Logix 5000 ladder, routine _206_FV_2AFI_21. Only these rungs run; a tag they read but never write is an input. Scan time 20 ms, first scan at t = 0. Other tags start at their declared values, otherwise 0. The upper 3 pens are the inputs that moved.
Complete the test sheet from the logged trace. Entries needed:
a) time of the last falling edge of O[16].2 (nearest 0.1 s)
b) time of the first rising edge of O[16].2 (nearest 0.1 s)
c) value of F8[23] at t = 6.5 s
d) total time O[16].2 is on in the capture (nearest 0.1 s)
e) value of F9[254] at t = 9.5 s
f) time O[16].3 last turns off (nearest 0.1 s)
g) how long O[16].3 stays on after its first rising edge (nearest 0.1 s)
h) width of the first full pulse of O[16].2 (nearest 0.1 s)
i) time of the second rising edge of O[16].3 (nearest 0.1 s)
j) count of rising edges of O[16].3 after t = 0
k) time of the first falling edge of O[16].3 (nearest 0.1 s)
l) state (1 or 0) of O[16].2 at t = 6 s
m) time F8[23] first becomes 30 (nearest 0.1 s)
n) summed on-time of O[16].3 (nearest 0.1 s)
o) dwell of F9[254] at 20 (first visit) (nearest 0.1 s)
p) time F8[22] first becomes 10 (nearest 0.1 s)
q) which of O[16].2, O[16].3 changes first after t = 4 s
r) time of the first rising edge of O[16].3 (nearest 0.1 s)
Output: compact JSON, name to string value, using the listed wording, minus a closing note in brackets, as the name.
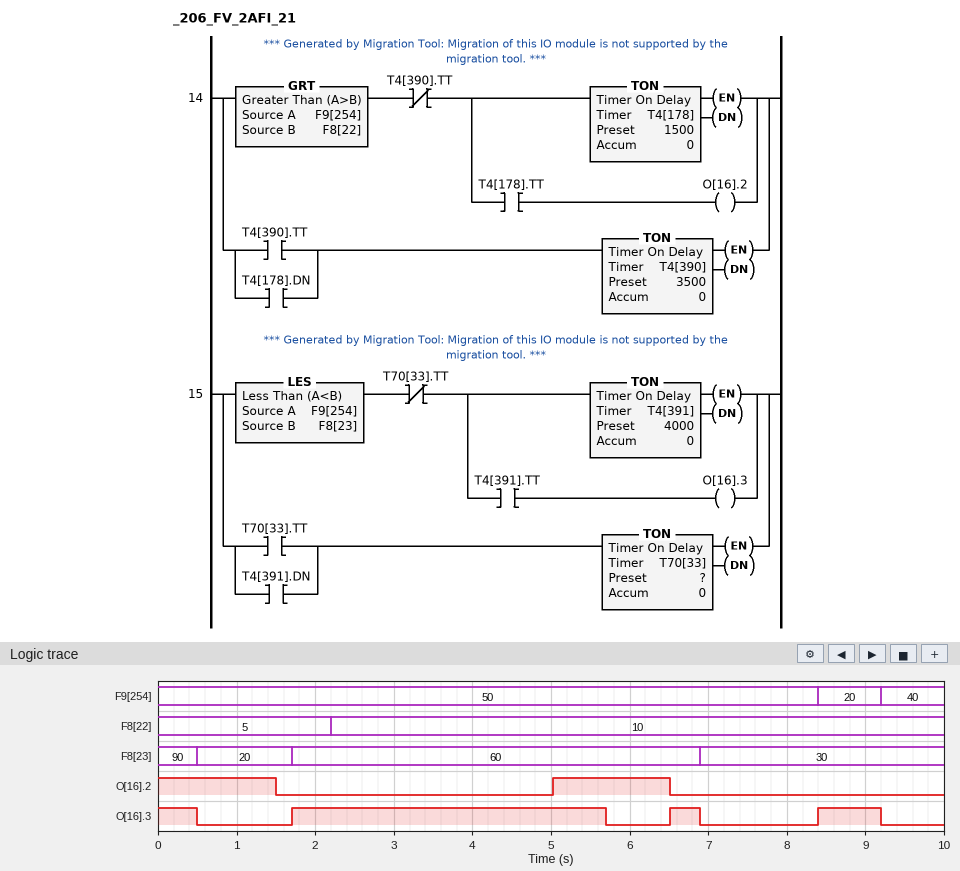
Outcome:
{"time of the last falling edge of O[16].2": "6.5 s", "time of the first rising edge of O[16].2": "5.0 s", "value of F8[23] at t = 6.5 s": "60", "total time O[16].2 is on in the capture": "3.0 s", "value of F9[254] at t = 9.5 s": "40", "time O[16].3 last turns off": "9.2 s", "how long O[16].3 stays on after its first rising edge": "4.0 s", "width of the first full pulse of O[16].2": "1.5 s", "time of the second rising edge of O[16].3": "6.5 s", "count of rising edges of O[16].3 after t = 0": "3", "time of the first falling edge of O[16].3": "0.5 s", "state (1 or 0) of O[16].2 at t = 6 s": "1", "time F8[23] first becomes 30": "6.9 s", "summed on-time of O[16].3": "5.7 s", "dwell of F9[254] at 20 (first visit)": "0.8 s", "time F8[22] first becomes 10": "2.2 s", "which of O[16].2, O[16].3 changes first after t = 4 s": "O[16].2", "time of the first rising edge of O[16].3": "1.7 s"}
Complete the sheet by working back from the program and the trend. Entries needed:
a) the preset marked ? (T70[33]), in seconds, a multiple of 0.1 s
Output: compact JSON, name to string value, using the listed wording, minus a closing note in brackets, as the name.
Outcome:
{"the preset marked ? (T70[33]), in seconds, a multiple of 0.1 s": "0.8 s"}
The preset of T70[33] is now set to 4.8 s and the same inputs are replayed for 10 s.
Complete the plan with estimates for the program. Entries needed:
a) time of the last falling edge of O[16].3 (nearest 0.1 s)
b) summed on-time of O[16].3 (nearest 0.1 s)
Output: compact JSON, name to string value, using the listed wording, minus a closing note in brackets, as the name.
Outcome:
{"time of the last falling edge of O[16].3": "5.7 s", "summed on-time of O[16].3": "4.5 s"}
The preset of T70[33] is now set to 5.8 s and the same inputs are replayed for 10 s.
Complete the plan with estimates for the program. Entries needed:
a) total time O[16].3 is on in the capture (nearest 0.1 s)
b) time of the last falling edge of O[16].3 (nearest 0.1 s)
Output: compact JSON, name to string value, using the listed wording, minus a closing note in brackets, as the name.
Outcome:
{"total time O[16].3 is on in the capture": "4.5 s", "time of the last falling edge of O[16].3": "5.7 s"}
